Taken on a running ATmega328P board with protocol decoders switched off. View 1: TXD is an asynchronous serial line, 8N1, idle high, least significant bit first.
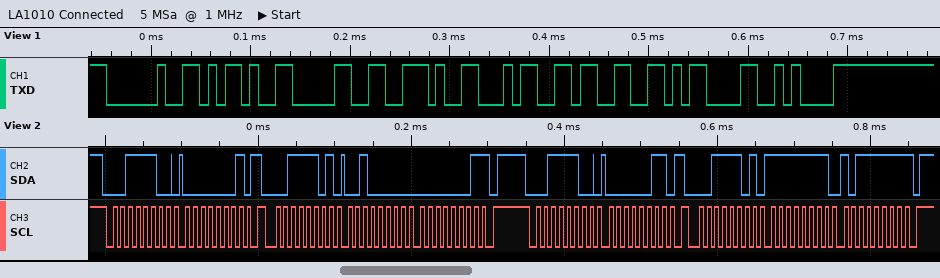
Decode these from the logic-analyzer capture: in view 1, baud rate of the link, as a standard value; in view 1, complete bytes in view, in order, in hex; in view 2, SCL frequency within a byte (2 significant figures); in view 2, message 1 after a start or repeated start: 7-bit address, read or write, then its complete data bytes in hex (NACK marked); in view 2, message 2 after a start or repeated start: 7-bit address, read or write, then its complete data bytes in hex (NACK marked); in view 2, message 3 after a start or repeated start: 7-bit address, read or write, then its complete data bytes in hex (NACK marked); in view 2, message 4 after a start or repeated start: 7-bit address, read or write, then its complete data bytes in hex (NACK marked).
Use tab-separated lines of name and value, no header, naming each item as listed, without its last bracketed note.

in view 1, baud rate of the link, as a standard value	115200 baud
in view 1, complete bytes in view, in order, in hex	20 2D 30 2E 34 33 0D 0A
in view 2, SCL frequency within a byte	100 kHz
in view 2, message 1 after a start or repeated start: 7-bit address, read or write, then its complete data bytes in hex	0x1E write: 01
in view 2, message 2 after a start or repeated start: 7-bit address, read or write, then its complete data bytes in hex	0x1E read: 20 01 NACK
in view 2, message 3 after a start or repeated start: 7-bit address, read or write, then its complete data bytes in hex	0x1E write: 03
in view 2, message 4 after a start or repeated start: 7-bit address, read or write, then its complete data bytes in hex	0x1E read: FF BF NACK
